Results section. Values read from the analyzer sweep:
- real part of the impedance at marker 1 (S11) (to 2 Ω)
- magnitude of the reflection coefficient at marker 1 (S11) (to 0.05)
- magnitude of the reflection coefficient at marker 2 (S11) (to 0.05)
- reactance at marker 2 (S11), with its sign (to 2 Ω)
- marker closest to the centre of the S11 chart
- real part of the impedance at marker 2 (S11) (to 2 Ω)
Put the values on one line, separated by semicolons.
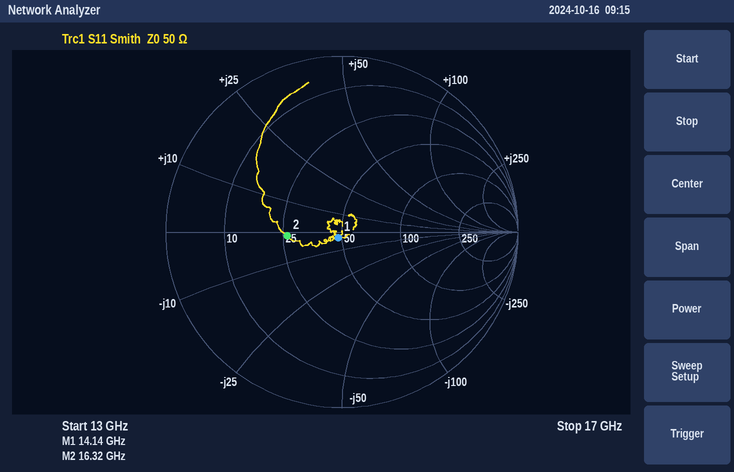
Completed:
48 Ω; 0.05; 0.30; -2 Ω; marker 1; 26 Ω
